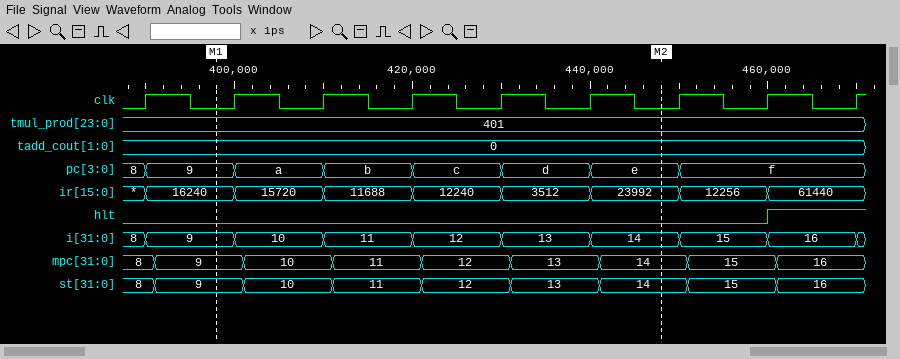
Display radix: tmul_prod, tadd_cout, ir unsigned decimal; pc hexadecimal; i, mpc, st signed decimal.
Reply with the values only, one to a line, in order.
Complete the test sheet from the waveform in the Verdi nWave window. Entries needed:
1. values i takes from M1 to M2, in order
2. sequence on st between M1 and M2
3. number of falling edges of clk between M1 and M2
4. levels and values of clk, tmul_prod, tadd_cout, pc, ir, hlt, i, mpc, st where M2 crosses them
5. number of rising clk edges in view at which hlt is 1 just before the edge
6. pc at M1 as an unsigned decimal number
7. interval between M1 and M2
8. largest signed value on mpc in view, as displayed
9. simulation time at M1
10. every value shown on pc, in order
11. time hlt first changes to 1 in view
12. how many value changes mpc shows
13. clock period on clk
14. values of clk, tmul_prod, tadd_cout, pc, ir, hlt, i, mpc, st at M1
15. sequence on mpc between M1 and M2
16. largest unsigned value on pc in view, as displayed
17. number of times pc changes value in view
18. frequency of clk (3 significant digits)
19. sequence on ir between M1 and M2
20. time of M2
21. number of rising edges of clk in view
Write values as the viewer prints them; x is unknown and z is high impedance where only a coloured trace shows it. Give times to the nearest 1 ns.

9, 10, 11, 12, 13, 14
9, 10, 11, 12, 13, 14
5
clk=0, tmul_prod=401, tadd_cout=0, pc=e, ir=23992, hlt=0, i=14, mpc=14, st=14
1
9
50 ns
16
398 ns
8, 9, a, b, c, d, e, f
460 ns
8
10 ns
clk=0, tmul_prod=401, tadd_cout=0, pc=9, ir=16240, hlt=0, i=9, mpc=9, st=9
9, 10, 11, 12, 13, 14
f
7
100 MHz
16240, 15720, 11688, 12240, 3512, 23992
448 ns
9
